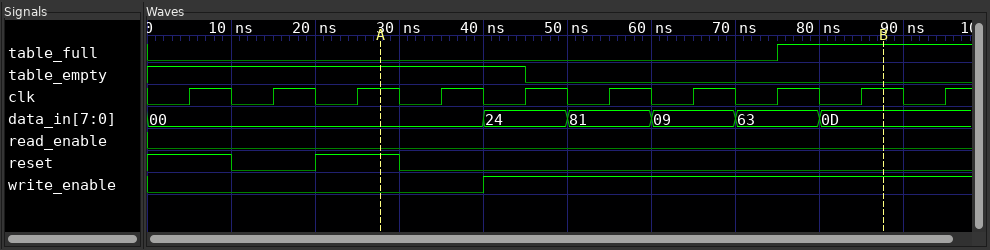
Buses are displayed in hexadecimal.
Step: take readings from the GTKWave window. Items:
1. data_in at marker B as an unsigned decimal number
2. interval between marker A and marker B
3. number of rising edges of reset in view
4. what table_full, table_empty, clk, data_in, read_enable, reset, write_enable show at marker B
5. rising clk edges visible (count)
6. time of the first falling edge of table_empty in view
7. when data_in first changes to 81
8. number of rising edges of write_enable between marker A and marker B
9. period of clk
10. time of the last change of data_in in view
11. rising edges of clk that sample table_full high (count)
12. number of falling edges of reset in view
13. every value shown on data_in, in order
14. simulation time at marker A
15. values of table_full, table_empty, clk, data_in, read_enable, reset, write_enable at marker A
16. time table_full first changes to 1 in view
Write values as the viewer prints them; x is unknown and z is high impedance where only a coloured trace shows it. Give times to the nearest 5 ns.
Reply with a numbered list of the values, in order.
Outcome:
1. 13
2. 60 ns
3. 1
4. table_full=1, table_empty=0, clk=1, data_in=0D, read_enable=0, reset=0, write_enable=1
5. 10
6. 45 ns
7. 50 ns
8. 1
9. 10 ns
10. 80 ns
11. 2
12. 2
13. 00, 24, 81, 09, 63, 0D
14. 30 ns
15. table_full=0, table_empty=1, clk=1, data_in=00, read_enable=0, reset=1, write_enable=0
16. 75 ns
